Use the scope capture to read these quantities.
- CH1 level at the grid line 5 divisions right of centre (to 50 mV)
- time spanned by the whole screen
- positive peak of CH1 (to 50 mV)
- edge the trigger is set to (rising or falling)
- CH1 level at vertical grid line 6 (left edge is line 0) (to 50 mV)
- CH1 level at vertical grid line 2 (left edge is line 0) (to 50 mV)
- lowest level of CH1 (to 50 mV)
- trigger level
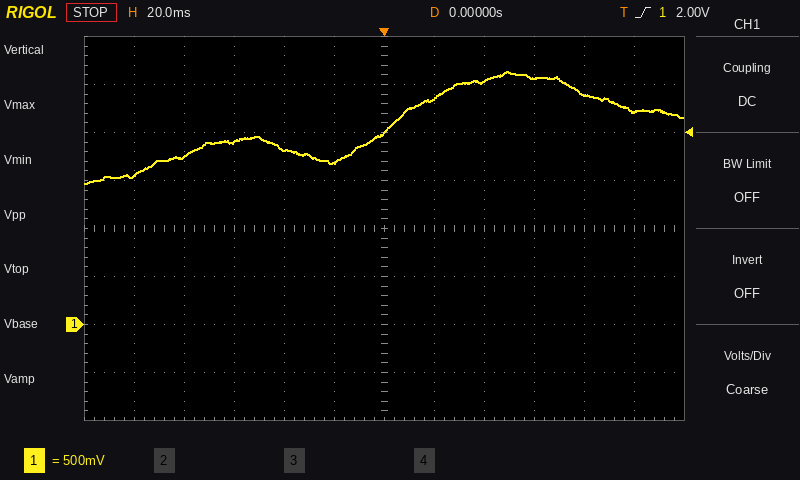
2.20 V
240 ms
2.65 V
rising
2.00 V
1.75 V
1.45 V
2.00 V
